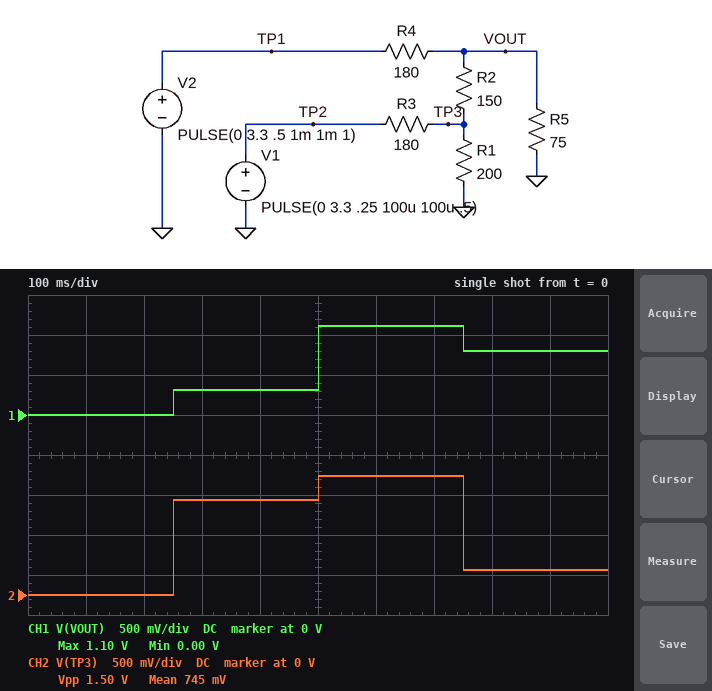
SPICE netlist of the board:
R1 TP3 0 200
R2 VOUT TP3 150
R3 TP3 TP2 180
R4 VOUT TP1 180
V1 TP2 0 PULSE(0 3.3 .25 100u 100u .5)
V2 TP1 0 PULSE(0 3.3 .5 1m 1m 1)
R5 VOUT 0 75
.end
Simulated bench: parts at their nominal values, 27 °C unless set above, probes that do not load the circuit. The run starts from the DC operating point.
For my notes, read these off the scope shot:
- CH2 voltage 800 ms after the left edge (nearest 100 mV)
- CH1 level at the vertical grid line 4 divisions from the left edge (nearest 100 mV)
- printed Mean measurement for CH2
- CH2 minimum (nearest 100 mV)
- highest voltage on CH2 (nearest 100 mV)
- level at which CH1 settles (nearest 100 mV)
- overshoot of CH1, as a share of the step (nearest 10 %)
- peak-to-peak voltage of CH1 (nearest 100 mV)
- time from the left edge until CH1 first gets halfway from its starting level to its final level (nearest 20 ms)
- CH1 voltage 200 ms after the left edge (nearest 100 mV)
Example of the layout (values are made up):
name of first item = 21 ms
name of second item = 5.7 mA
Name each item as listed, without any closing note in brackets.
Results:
CH2 voltage 800 ms after the left edge = 300 mV
CH1 level at the vertical grid line 4 divisions from the left edge = 300 mV
printed Mean measurement for CH2 = 745 mV
CH2 minimum = 0 V
highest voltage on CH2 = 1.5 V
level at which CH1 settles = 800 mV
overshoot of CH1, as a share of the step = 40 %
peak-to-peak voltage of CH1 = 1.1 V
time from the left edge until CH1 first gets halfway from its starting level to its final level = 500 ms
CH1 voltage 200 ms after the left edge = 0 V
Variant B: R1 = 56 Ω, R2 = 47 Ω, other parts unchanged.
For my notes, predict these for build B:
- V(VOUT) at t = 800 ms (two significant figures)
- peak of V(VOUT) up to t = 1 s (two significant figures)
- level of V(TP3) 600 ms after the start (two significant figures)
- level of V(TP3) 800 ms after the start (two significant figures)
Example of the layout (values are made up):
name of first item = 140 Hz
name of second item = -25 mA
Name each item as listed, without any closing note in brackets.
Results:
V(VOUT) at t = 800 ms = 610 mV
peak of V(VOUT) up to t = 1 s = 900 mV
level of V(TP3) 600 ms after the start = 840 mV
level of V(TP3) 800 ms after the start = 290 mV
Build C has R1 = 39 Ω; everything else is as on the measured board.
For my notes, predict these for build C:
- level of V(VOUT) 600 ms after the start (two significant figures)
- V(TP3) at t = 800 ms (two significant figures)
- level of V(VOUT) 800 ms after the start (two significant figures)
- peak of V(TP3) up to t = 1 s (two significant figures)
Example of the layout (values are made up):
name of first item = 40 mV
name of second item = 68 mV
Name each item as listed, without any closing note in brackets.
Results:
level of V(VOUT) 600 ms after the start = 880 mV
V(TP3) at t = 800 ms = 130 mV
level of V(VOUT) 800 ms after the start = 750 mV
peak of V(TP3) up to t = 1 s = 640 mV
